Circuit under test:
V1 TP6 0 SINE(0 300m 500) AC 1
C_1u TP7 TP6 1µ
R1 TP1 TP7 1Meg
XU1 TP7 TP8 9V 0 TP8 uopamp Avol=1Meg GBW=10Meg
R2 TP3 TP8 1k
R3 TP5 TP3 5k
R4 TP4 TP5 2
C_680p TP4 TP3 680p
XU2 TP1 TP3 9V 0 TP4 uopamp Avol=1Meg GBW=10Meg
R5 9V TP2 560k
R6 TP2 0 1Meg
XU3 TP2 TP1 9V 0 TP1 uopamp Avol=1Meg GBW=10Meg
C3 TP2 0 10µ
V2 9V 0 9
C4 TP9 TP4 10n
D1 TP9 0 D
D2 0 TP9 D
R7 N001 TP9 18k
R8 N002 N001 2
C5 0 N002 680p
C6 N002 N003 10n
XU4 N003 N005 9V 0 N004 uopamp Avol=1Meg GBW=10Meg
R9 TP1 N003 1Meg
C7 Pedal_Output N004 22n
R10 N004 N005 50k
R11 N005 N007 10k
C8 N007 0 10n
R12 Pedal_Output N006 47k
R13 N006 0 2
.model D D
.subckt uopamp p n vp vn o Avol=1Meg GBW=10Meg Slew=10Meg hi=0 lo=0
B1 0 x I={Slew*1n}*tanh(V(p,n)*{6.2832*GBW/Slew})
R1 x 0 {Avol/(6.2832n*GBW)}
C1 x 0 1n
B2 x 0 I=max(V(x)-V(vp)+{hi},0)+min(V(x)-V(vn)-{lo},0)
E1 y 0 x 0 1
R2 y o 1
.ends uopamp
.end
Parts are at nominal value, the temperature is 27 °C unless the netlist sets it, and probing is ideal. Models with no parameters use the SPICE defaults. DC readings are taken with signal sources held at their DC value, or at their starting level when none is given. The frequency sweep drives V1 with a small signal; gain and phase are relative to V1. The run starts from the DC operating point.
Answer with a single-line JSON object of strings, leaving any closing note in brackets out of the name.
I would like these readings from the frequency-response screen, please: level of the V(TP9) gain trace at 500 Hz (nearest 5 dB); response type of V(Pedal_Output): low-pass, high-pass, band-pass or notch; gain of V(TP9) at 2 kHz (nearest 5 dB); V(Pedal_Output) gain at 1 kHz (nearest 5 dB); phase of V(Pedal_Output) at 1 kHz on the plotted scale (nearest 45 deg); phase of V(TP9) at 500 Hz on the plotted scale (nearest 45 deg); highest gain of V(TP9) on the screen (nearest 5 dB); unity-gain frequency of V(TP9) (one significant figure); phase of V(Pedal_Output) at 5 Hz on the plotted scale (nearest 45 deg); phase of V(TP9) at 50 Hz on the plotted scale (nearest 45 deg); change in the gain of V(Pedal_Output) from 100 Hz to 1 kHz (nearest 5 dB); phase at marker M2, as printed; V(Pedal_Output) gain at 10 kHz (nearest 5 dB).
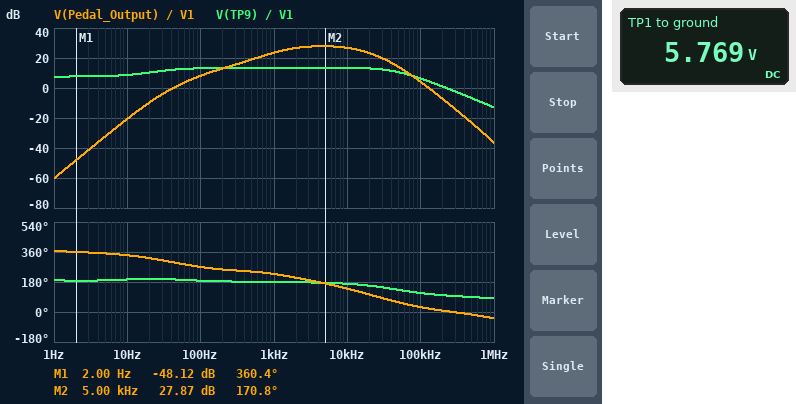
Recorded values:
{"level of the V(TP9) gain trace at 500 Hz": "15 dB", "response type of V(Pedal_Output): low-pass, high-pass, band-pass or notch": "band-pass", "gain of V(TP9) at 2 kHz": "15 dB", "V(Pedal_Output) gain at 1 kHz": "25 dB", "phase of V(Pedal_Output) at 1 kHz on the plotted scale": "225 deg", "phase of V(TP9) at 500 Hz on the plotted scale": "180 deg", "highest gain of V(TP9) on the screen": "15 dB", "unity-gain frequency of V(TP9)": "200 kHz", "phase of V(Pedal_Output) at 5 Hz on the plotted scale": "360 deg", "phase of V(TP9) at 50 Hz on the plotted scale": "180 deg", "change in the gain of V(Pedal_Output) from 100 Hz to 1 kHz": "15 dB", "phase at marker M2, as printed": "170.8 deg", "V(Pedal_Output) gain at 10 kHz": "25 dB"}
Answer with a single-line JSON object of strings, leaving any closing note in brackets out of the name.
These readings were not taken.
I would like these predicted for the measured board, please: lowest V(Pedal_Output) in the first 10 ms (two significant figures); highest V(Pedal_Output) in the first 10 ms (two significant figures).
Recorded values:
{"lowest V(Pedal_Output) in the first 10 ms": "-2.2 V", "highest V(Pedal_Output) in the first 10 ms": "2.2 V"}
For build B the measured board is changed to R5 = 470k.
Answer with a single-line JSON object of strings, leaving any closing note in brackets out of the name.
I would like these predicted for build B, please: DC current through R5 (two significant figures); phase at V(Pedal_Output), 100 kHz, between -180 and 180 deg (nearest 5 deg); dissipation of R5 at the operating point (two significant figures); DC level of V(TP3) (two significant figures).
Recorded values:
{"DC current through R5": "6.1 µA", "phase at V(Pedal_Output), 100 kHz, between -180 and 180 deg": "30 deg", "dissipation of R5 at the operating point": "18 µW", "DC level of V(TP3)": "6.1 V"}
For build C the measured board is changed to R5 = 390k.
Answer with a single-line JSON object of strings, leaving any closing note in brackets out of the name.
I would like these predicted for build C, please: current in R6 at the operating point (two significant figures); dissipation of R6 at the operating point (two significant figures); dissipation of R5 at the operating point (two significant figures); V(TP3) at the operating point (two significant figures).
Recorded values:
{"current in R6 at the operating point": "6.5 µA", "dissipation of R6 at the operating point": "42 µW", "dissipation of R5 at the operating point": "16 µW", "V(TP3) at the operating point": "6.5 V"}
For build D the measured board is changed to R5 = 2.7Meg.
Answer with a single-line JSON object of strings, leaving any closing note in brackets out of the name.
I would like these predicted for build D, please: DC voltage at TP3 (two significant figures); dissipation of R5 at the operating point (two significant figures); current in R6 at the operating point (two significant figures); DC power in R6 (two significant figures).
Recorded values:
{"DC voltage at TP3": "2.4 V", "dissipation of R5 at the operating point": "16 µW", "current in R6 at the operating point": "2.4 µA", "DC power in R6": "5.9 µW"}
